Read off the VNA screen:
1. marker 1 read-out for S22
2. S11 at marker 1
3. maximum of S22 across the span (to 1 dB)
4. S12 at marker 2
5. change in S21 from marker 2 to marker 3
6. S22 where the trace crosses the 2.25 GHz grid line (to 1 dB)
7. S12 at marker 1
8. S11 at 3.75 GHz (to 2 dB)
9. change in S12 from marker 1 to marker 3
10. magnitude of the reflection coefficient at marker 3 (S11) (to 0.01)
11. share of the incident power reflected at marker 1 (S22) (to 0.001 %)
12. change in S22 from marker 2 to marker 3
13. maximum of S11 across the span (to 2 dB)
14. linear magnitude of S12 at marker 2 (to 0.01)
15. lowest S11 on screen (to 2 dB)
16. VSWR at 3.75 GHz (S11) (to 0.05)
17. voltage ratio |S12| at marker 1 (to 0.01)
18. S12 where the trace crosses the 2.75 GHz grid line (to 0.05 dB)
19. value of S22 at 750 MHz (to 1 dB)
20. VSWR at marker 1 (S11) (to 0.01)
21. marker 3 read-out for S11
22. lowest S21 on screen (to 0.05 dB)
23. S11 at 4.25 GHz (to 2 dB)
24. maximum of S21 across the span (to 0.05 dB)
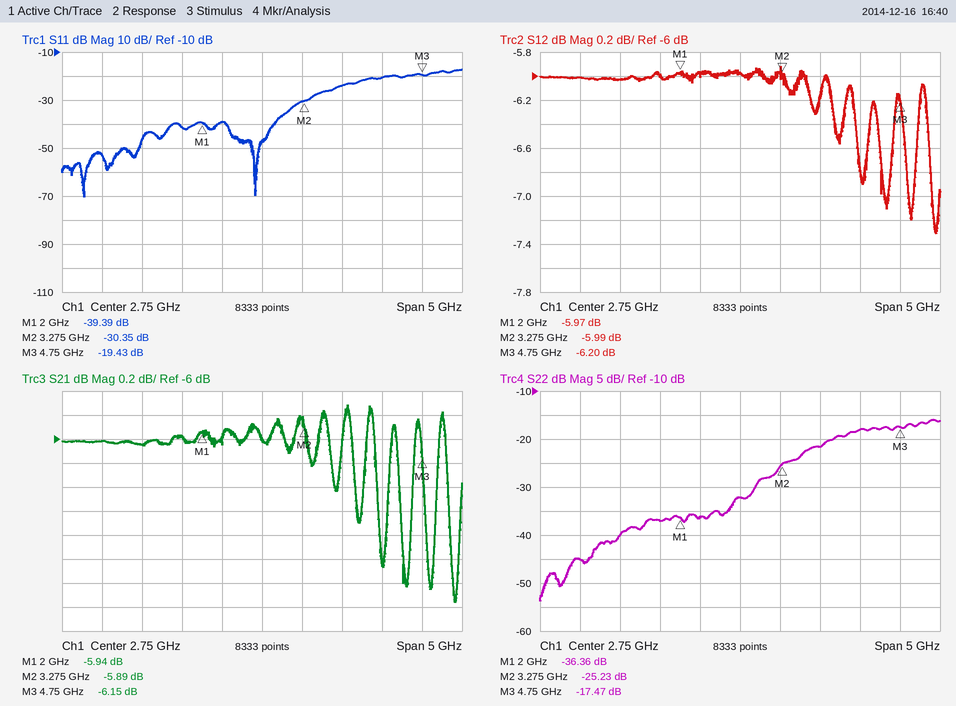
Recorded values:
-36.36 dB
-39.39 dB
-16 dB
-5.99 dB
-0.26 dB
-36 dB
-5.97 dB
-24 dB
-0.23 dB
0.11
0.023 %
7.76 dB
-18 dB
0.50
-70 dB
1.15
0.50
-6.00 dB
-45 dB
1.02
-19.43 dB
-7.35 dB
-20 dB
-5.70 dB
